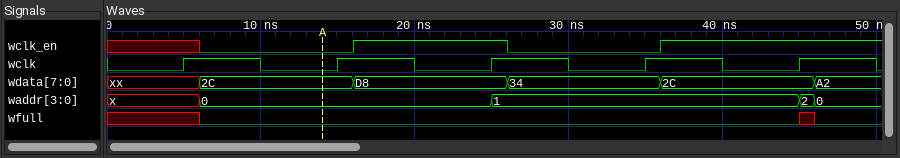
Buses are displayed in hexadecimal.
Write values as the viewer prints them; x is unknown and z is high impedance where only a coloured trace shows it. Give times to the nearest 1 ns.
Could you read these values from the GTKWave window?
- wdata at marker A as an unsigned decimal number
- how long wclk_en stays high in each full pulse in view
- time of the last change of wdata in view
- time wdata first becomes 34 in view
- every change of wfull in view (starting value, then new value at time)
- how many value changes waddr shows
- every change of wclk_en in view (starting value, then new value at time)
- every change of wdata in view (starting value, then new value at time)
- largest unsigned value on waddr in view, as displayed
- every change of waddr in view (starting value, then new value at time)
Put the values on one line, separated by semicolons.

44; 10 ns; 46 ns; 26 ns; x, 0 at 6 ns, x at 45 ns, 0 at 46 ns; 4; x, 0 at 6 ns, 1 at 16 ns, 0 at 26 ns, 1 at 36 ns; xx, 2C at 6 ns, D8 at 16 ns, 34 at 26 ns, 2C at 36 ns, A2 at 46 ns; 2; x, 0 at 6 ns, 1 at 25 ns, 2 at 45 ns, 0 at 46 ns
